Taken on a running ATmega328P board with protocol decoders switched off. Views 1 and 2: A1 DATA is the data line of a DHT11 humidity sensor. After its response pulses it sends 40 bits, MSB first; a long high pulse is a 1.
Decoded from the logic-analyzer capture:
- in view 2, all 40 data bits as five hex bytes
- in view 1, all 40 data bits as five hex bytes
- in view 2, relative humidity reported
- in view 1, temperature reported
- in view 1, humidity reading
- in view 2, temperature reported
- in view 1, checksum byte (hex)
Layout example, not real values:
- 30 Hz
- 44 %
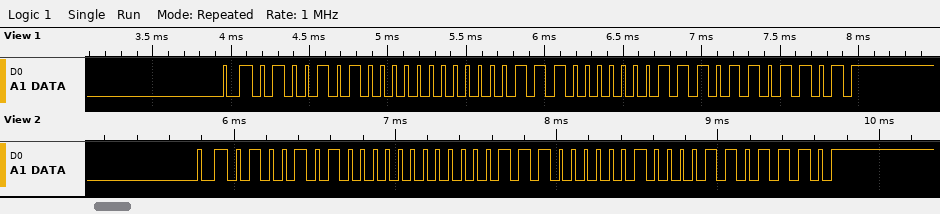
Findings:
- 4A 00 1C 08 6E
- 4A 00 1C 07 6D
- 74 %
- 28.7 °C
- 74 %
- 28.8 °C
- 0x6D
